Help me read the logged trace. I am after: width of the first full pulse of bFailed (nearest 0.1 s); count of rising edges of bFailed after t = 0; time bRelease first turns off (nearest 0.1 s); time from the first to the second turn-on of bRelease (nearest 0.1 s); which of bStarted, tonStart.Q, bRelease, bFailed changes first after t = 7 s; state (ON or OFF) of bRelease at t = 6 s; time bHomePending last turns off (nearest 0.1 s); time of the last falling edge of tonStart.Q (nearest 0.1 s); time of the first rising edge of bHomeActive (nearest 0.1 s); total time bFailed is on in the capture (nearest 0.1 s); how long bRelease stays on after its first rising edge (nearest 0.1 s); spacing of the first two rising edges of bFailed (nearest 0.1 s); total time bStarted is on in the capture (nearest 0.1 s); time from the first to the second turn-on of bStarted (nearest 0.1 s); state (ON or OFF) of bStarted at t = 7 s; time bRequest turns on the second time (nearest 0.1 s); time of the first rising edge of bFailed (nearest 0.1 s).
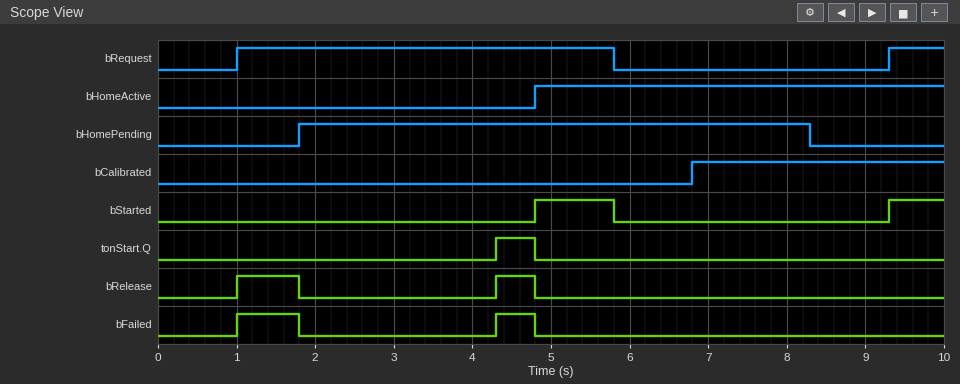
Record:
0.8 s
2
1.8 s
3.3 s
bStarted
OFF
8.3 s
4.8 s
4.8 s
1.3 s
0.8 s
3.3 s
1.7 s
4.5 s
OFF
9.3 s
1.0 s
